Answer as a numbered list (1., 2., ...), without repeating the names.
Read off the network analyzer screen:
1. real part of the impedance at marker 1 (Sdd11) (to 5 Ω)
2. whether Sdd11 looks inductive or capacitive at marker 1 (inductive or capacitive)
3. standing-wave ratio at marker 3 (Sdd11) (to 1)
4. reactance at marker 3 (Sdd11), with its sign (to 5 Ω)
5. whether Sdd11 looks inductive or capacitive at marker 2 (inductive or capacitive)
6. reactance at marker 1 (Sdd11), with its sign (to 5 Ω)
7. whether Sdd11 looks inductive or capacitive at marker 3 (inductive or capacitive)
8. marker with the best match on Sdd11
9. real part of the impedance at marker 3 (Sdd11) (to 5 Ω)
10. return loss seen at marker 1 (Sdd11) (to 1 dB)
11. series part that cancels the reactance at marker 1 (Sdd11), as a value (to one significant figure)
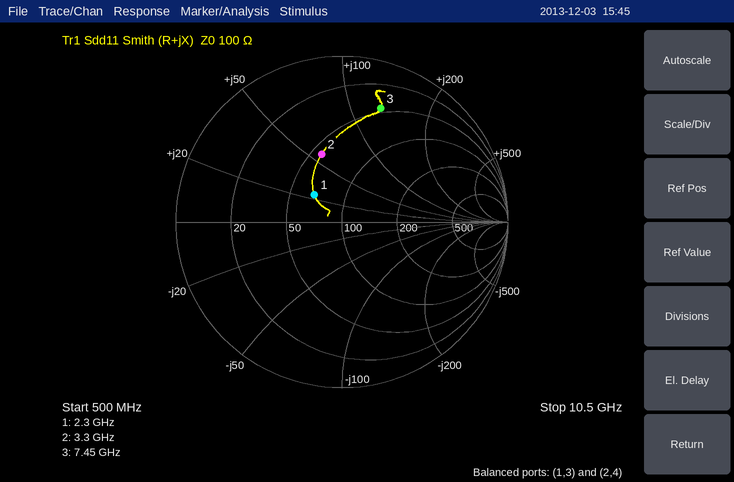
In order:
1. 70 Ω
2. inductive
3. 6
4. +130 Ω
5. inductive
6. +25 Ω
7. inductive
8. marker 1
9. 45 Ω
10. 13 dB
11. 3 pF
